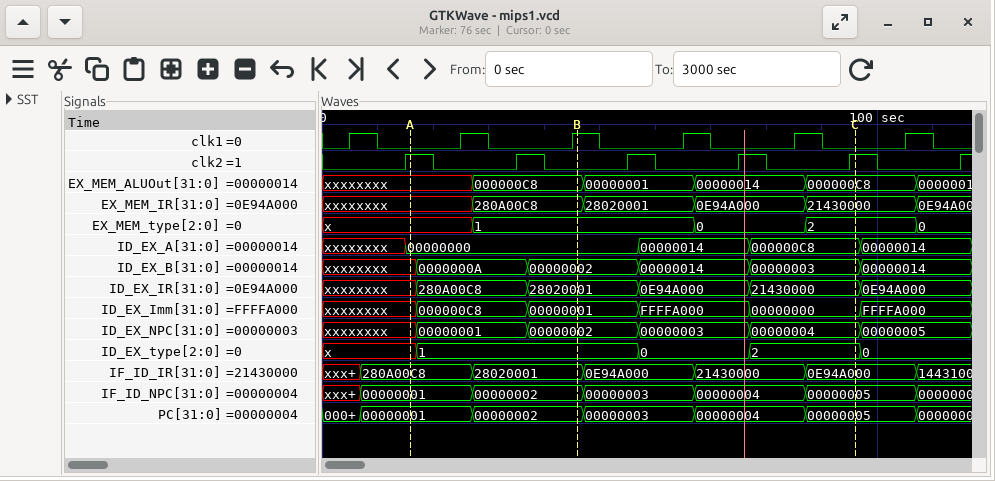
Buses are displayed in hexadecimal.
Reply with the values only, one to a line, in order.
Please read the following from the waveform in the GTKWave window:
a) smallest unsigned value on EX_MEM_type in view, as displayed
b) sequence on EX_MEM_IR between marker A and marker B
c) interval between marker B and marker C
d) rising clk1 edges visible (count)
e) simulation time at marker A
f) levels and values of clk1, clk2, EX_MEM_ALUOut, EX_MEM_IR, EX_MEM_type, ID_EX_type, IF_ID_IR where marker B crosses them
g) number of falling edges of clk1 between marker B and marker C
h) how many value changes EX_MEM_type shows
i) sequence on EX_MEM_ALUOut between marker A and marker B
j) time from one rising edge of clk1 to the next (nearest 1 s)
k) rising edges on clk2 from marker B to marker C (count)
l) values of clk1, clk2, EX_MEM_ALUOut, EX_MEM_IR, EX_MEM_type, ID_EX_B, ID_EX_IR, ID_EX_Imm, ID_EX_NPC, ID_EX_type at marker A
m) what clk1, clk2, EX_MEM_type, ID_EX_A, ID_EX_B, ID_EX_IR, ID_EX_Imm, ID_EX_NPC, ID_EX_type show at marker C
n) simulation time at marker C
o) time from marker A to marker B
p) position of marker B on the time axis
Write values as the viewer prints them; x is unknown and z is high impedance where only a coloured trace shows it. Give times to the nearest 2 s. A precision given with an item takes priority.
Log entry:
0
xxxxxxxx, 280A00C8
50 s
6
16 s
clk1=1, clk2=0, EX_MEM_ALUOut=000000C8, EX_MEM_IR=280A00C8, EX_MEM_type=1, ID_EX_type=1, IF_ID_IR=28020001
3
4
xxxxxxxx, 000000C8
20 s
3
clk1=0, clk2=1, EX_MEM_ALUOut=xxxxxxxx, EX_MEM_IR=xxxxxxxx, EX_MEM_type=x, ID_EX_B=xxxxxxxx, ID_EX_IR=xxxxxxxx, ID_EX_Imm=xxxxxxxx, ID_EX_NPC=xxxxxxxx, ID_EX_type=x
clk1=0, clk2=1, EX_MEM_type=2, ID_EX_A=000000C8, ID_EX_B=00000003, ID_EX_IR=21430000, ID_EX_Imm=00000000, ID_EX_NPC=00000004, ID_EX_type=2
96 s
30 s
46 s
